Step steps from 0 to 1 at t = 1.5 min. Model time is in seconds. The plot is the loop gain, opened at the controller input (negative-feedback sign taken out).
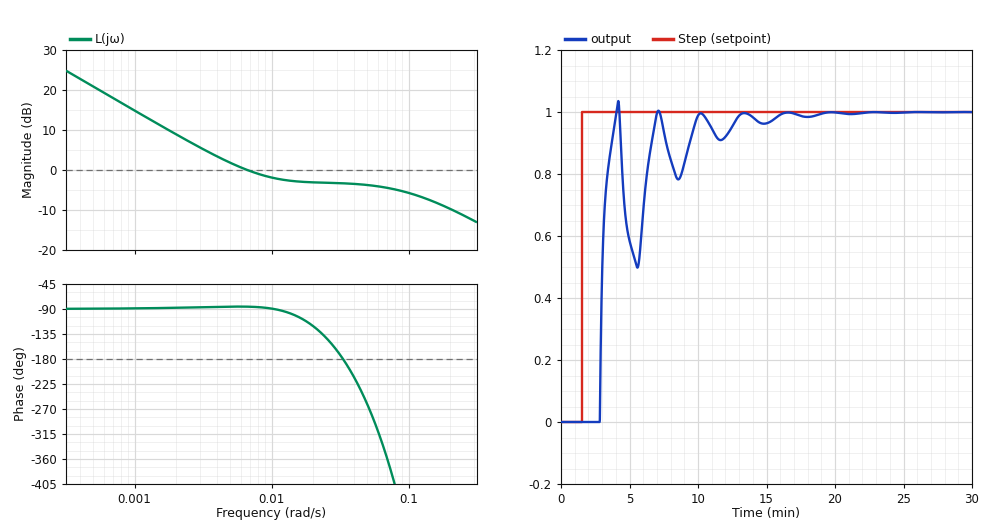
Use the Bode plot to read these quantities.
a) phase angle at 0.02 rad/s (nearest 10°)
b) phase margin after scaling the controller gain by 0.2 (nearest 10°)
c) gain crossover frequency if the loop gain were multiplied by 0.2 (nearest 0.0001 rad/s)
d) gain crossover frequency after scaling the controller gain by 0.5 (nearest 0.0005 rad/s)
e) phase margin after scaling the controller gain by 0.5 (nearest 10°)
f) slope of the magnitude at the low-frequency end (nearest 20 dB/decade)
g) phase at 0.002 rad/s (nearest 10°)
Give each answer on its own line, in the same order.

-120°
90°
0.0011 rad/s
0.0030 rad/s
90°
-20 dB/decade
-90°
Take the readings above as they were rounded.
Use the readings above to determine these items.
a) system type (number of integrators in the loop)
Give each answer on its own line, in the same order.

1
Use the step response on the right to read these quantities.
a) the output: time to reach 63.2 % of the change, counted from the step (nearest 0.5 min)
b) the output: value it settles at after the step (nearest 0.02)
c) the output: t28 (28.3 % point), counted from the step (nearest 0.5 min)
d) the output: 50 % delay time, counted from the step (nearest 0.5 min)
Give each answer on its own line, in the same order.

1.5 min
1.00
1.5 min
1.5 min
